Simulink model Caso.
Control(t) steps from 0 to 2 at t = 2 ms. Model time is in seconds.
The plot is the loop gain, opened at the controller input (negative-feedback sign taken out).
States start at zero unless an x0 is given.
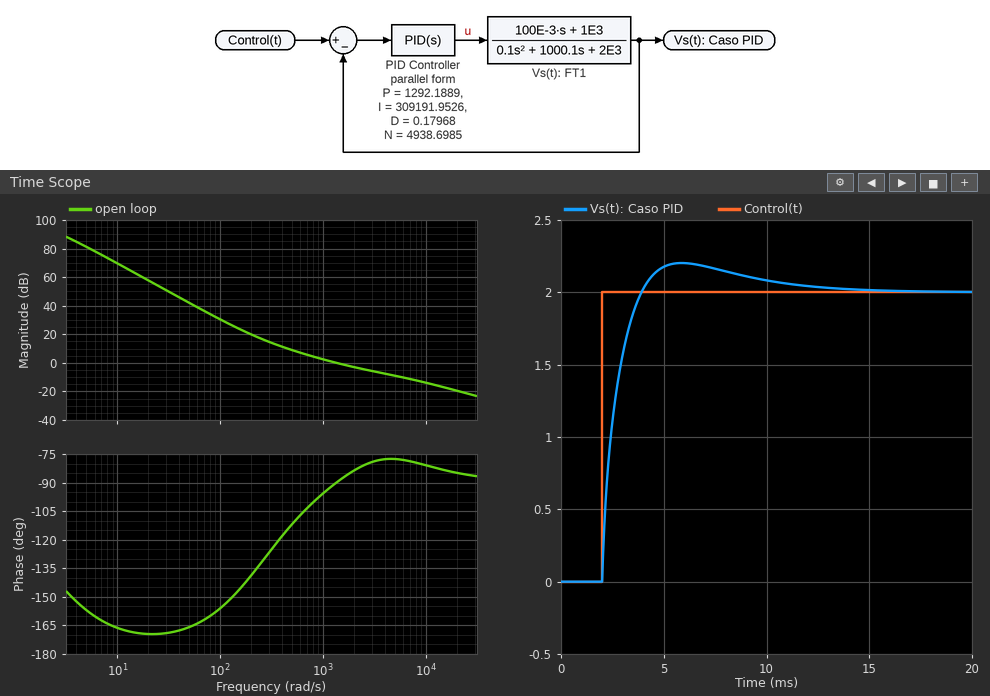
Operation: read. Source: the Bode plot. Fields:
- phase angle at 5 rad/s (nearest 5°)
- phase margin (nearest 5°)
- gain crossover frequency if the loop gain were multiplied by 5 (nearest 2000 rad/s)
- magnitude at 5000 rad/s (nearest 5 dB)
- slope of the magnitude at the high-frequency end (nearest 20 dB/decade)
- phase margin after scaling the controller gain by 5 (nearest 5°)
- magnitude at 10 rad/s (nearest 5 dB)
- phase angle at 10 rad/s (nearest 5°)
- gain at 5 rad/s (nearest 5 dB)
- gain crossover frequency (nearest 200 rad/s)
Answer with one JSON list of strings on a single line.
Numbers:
["-155°", "90°", "10000 rad/s", "-10 dB", "-20 dB/decade", "100°", "70 dB", "-165°", "80 dB", "1400 rad/s"]
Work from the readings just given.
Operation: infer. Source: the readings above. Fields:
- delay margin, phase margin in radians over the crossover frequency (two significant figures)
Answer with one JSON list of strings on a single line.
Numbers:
["0.0011 s"]
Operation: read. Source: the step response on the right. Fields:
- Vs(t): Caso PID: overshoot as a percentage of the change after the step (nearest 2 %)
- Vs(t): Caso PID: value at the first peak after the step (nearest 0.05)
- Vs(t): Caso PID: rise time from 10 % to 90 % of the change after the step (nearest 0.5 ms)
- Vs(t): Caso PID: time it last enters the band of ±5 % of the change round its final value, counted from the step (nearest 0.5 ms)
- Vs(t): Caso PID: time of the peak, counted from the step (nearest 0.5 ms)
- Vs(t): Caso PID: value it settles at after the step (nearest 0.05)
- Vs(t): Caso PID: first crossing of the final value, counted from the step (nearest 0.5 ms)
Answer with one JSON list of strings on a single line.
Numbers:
["10 %", "2.20", "1.5 ms", "7.5 ms", "4.0 ms", "2.00", "2.0 ms"]
